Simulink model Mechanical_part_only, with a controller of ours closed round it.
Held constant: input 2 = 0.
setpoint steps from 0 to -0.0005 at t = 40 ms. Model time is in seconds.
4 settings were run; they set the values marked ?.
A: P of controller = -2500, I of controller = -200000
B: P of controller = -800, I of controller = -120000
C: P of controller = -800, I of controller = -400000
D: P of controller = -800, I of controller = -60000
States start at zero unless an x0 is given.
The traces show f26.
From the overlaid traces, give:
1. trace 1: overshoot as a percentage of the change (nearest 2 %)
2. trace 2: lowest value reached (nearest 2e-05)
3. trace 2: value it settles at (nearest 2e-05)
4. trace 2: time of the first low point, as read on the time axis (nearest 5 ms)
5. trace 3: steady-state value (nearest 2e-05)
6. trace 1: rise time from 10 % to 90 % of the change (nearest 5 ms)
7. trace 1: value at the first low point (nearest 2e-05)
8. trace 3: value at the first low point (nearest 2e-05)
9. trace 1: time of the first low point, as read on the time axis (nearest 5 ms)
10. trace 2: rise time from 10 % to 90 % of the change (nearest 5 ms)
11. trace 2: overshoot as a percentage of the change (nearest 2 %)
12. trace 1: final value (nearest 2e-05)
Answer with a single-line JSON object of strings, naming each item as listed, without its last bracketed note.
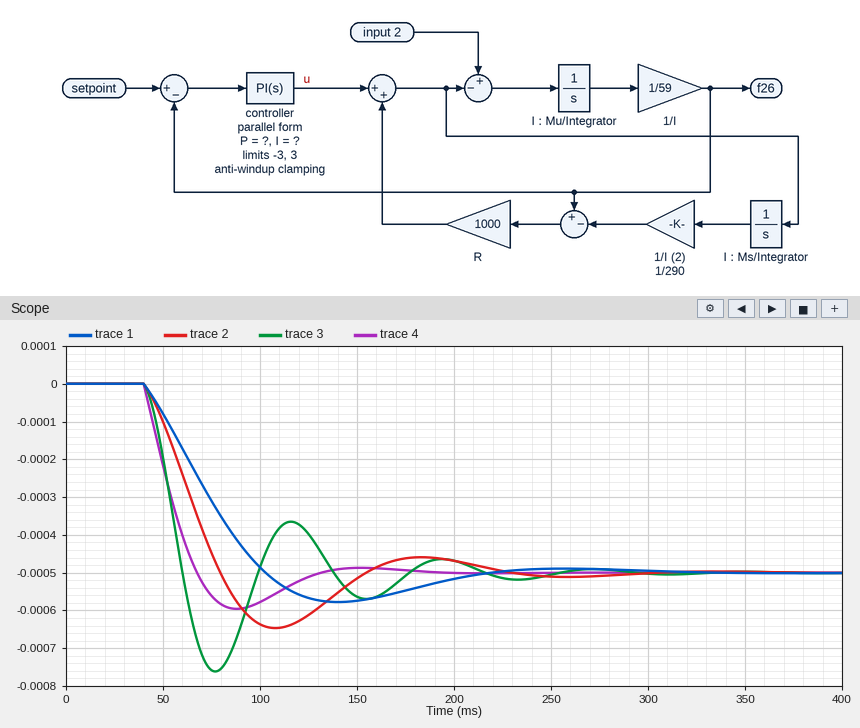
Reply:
{"trace 1: overshoot as a percentage of the change": "16 %", "trace 2: lowest value reached": "-0.00064", "trace 2: value it settles at": "-0.00050", "trace 2: time of the first low point, as read on the time axis": "110 ms", "trace 3: steady-state value": "-0.00050", "trace 1: rise time from 10 % to 90 % of the change": "45 ms", "trace 1: value at the first low point": "-0.00058", "trace 3: value at the first low point": "-0.00076", "trace 1: time of the first low point, as read on the time axis": "140 ms", "trace 2: rise time from 10 % to 90 % of the change": "30 ms", "trace 2: overshoot as a percentage of the change": "30 %", "trace 1: final value": "-0.00050"}
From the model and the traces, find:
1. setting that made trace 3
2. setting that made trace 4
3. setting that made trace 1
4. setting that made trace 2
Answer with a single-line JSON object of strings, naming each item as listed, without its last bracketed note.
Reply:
{"setting that made trace 3": "C", "setting that made trace 4": "A", "setting that made trace 1": "D", "setting that made trace 2": "B"}
